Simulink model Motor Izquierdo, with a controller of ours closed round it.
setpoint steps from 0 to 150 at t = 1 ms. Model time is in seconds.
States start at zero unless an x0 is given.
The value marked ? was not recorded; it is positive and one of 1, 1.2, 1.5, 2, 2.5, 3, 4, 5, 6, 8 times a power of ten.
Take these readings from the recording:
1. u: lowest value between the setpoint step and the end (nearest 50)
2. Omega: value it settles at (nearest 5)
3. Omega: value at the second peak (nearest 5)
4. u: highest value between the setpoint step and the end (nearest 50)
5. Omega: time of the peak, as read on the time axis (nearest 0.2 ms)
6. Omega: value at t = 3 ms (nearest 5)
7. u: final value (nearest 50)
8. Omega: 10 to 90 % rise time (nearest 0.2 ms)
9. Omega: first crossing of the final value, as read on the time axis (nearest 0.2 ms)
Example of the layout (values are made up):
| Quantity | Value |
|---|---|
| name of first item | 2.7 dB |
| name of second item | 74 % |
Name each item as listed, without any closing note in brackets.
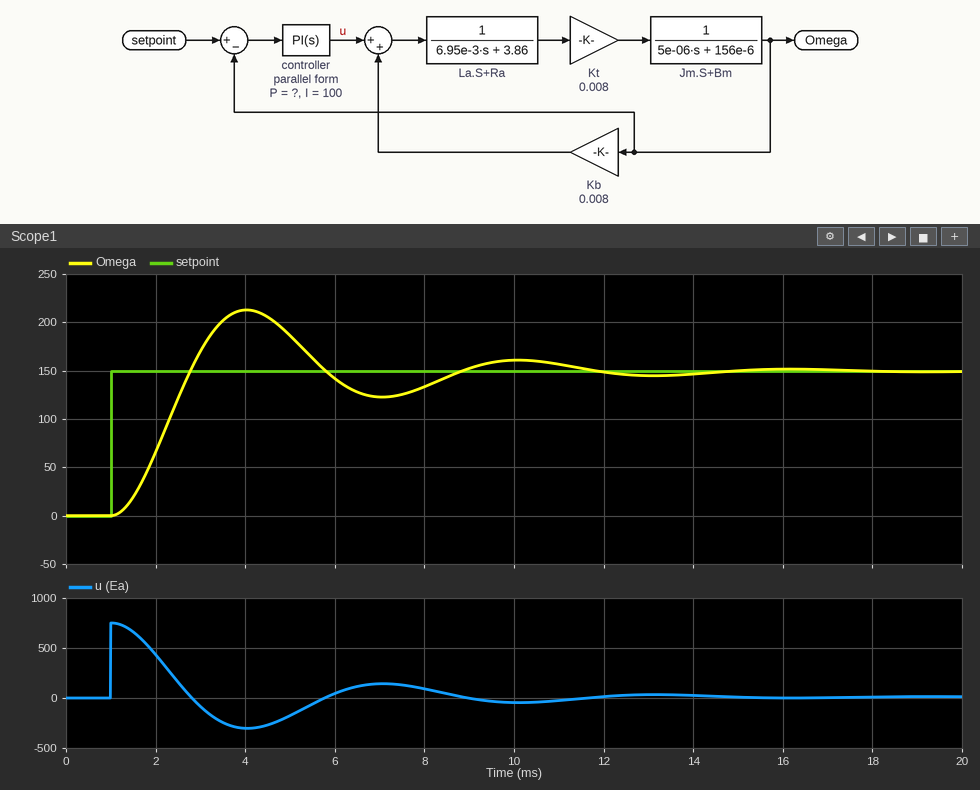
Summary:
| Quantity | Value |
|---|---|
| u: lowest value between the setpoint step and the end | -300 |
| Omega: value it settles at | 150 |
| Omega: value at the second peak | 160 |
| u: highest value between the setpoint step and the end | 750 |
| Omega: time of the peak, as read on the time axis | 4.0 ms |
| Omega: value at t = 3 ms | 170 |
| u: final value | 0 |
| Omega: 10 to 90 % rise time | 1.2 ms |
| Omega: first crossing of the final value, as read on the time axis | 2.8 ms |
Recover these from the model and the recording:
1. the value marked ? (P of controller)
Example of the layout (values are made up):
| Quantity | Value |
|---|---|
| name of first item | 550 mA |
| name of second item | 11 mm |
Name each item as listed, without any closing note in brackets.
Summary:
| Quantity | Value |
|---|---|
| the value marked ? | 5 |
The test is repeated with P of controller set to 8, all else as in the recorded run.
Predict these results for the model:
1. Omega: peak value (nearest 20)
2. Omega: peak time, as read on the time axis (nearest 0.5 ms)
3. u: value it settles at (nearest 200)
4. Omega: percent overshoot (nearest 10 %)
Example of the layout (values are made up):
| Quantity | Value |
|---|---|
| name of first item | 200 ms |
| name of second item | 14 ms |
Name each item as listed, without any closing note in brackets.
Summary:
| Quantity | Value |
|---|---|
| Omega: peak value | 220 |
| Omega: peak time, as read on the time axis | 3.5 ms |
| u: value it settles at | 0 |
| Omega: percent overshoot | 50 % |
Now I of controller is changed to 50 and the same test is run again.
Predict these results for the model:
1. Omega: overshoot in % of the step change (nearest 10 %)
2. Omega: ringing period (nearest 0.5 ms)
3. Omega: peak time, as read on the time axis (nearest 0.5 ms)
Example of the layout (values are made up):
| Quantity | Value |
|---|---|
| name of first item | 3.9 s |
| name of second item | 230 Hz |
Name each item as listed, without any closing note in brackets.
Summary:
| Quantity | Value |
|---|---|
| Omega: overshoot in % of the step change | 40 % |
| Omega: ringing period | 6.0 ms |
| Omega: peak time, as read on the time axis | 4.0 ms |
